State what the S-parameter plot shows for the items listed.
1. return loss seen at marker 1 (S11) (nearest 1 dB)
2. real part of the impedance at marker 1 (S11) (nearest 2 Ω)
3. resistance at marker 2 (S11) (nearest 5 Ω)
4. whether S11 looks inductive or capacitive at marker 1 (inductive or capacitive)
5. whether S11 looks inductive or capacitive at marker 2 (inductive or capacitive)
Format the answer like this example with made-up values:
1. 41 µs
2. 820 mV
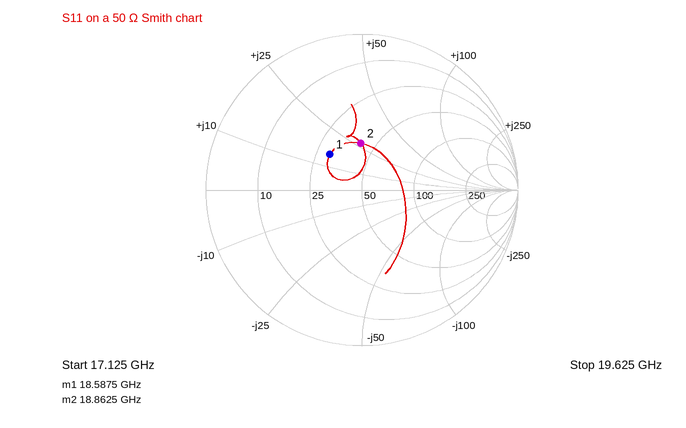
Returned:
1. 10 dB
2. 30 Ω
3. 40 Ω
4. inductive
5. inductive
